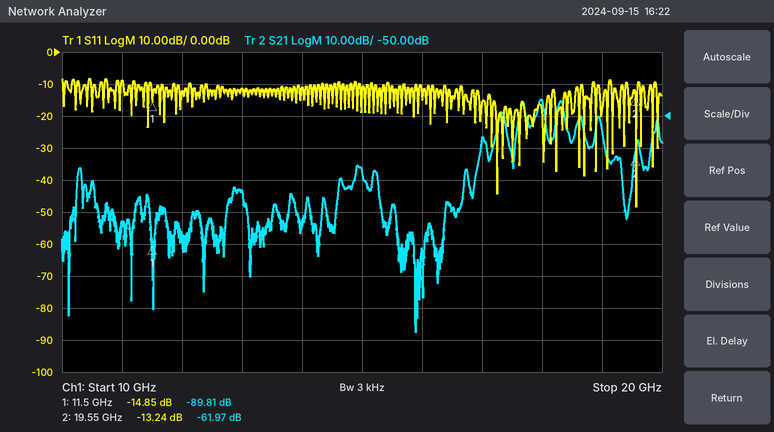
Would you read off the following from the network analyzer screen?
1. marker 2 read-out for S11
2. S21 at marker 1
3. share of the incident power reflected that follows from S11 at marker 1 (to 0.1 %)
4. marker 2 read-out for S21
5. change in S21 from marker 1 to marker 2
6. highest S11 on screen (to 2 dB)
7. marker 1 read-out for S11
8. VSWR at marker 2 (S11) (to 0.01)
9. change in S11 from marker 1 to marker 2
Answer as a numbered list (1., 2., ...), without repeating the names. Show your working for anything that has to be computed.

1. -13.24 dB
2. -89.81 dB
3. 10^(-14.85/10) ≈ 3.3 %
4. -61.97 dB
5. -61.97 − (-89.81) = 27.84 dB
6. -8 dB
7. -14.85 dB
8. (1 + 0.2178)/(1 − 0.2178) ≈ 1.56
9. -13.24 − (-14.85) = 1.61 dB
